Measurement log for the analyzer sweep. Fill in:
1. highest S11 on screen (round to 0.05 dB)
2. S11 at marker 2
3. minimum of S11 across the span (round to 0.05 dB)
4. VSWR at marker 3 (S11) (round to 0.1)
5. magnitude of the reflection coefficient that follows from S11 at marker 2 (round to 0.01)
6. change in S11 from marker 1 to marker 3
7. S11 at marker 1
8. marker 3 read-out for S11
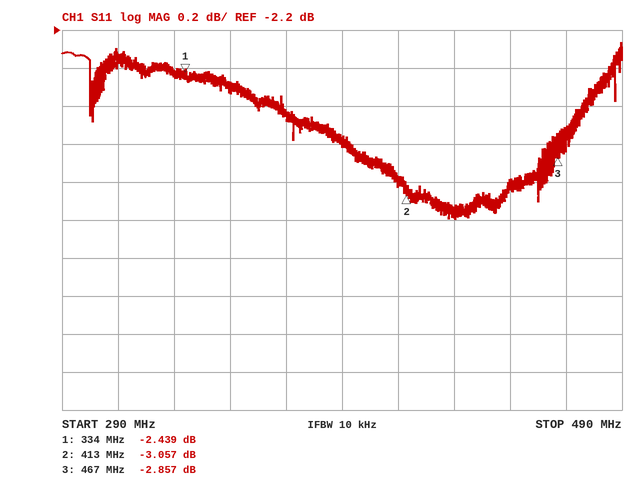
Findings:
-2.25 dB
-3.057 dB
-3.20 dB
6.1
0.70
-0.418 dB
-2.439 dB
-2.857 dB
